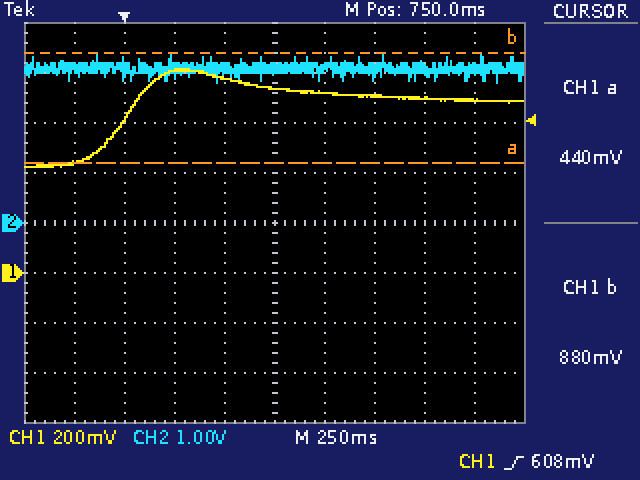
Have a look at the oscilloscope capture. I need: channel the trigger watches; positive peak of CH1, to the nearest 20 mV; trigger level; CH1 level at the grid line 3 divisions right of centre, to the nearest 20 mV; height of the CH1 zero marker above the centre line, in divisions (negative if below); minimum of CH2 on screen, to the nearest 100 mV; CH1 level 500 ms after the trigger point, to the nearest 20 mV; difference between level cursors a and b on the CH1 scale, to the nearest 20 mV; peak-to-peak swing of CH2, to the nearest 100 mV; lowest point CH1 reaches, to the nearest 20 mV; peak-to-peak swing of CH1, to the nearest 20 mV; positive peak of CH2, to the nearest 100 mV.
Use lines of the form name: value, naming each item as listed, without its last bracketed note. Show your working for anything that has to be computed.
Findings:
channel the trigger watches: CH1
positive peak of CH1, to the nearest 20 mV: 820 mV
trigger level: 608 mV
CH1 level at the grid line 3 divisions right of centre, to the nearest 20 mV: 700 mV
height of the CH1 zero marker above the centre line, in divisions: -1.0 div
minimum of CH2 on screen, to the nearest 100 mV: 2.8 V
CH1 level 500 ms after the trigger point, to the nearest 20 mV: 780 mV
difference between level cursors a and b on the CH1 scale, to the nearest 20 mV: 440 mV
peak-to-peak swing of CH2, to the nearest 100 mV: 3.4 V − (2.8 V) = 600 mV
lowest point CH1 reaches, to the nearest 20 mV: 420 mV
peak-to-peak swing of CH1, to the nearest 20 mV: 820 mV − (420 mV) = 400 mV
positive peak of CH2, to the nearest 100 mV: 3.4 V
